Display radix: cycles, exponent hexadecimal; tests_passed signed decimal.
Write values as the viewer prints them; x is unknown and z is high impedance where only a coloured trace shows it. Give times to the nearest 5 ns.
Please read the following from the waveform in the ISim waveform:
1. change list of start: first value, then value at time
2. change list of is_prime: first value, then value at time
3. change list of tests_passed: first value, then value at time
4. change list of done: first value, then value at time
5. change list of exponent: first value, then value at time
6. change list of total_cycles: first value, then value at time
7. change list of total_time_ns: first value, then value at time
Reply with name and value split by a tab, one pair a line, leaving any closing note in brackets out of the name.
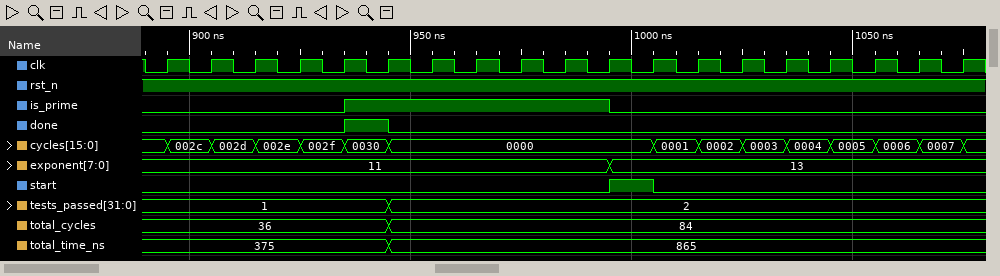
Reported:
change list of start: first value, then value at time	0, 1 at 995 ns, 0 at 1005 ns
change list of is_prime: first value, then value at time	0, 1 at 935 ns, 0 at 995 ns
change list of tests_passed: first value, then value at time	1, 2 at 945 ns
change list of done: first value, then value at time	0, 1 at 935 ns, 0 at 945 ns
change list of exponent: first value, then value at time	11, 13 at 995 ns
change list of total_cycles: first value, then value at time	36, 84 at 945 ns
change list of total_time_ns: first value, then value at time	375, 865 at 945 ns
